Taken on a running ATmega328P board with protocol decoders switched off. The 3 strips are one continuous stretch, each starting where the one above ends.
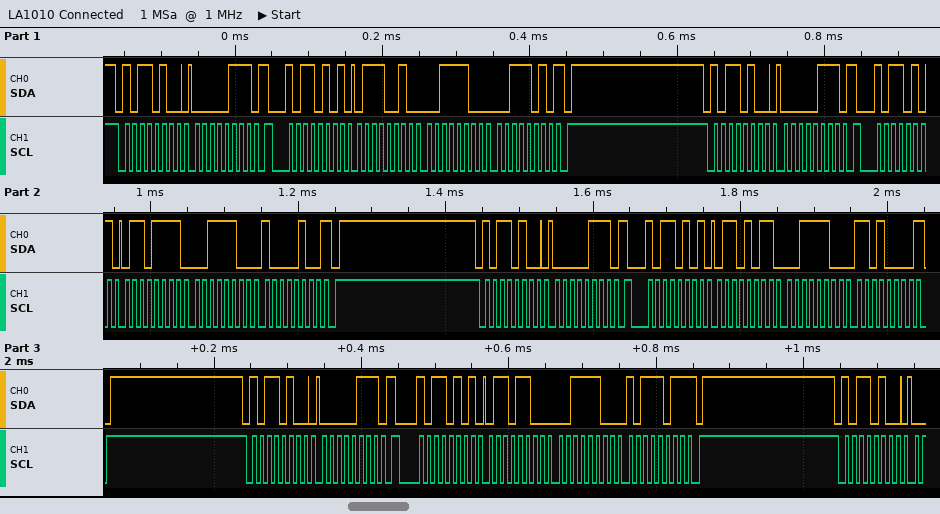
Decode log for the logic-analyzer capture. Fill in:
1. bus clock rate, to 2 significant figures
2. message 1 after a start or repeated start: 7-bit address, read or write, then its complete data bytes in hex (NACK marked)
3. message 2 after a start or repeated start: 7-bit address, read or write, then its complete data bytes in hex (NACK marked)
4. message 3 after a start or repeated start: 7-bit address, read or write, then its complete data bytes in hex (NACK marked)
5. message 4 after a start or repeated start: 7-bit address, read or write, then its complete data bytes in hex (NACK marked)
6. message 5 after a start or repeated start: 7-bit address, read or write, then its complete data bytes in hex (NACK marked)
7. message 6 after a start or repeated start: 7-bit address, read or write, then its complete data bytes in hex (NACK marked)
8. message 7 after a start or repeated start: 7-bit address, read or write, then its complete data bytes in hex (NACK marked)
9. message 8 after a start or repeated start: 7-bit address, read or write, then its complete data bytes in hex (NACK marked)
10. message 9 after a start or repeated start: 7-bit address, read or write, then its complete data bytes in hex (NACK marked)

100 kHz
0x5A write: 07
0x5A read: 72 3C 3A NACK
0x5A write: 07
0x5A read: 6F 3C 84 NACK
0x5A write: 07
0x5A read: 6B 3C D0 NACK
0x5A write: 07
0x5A read: 6C 3C BB NACK
0x5A write
